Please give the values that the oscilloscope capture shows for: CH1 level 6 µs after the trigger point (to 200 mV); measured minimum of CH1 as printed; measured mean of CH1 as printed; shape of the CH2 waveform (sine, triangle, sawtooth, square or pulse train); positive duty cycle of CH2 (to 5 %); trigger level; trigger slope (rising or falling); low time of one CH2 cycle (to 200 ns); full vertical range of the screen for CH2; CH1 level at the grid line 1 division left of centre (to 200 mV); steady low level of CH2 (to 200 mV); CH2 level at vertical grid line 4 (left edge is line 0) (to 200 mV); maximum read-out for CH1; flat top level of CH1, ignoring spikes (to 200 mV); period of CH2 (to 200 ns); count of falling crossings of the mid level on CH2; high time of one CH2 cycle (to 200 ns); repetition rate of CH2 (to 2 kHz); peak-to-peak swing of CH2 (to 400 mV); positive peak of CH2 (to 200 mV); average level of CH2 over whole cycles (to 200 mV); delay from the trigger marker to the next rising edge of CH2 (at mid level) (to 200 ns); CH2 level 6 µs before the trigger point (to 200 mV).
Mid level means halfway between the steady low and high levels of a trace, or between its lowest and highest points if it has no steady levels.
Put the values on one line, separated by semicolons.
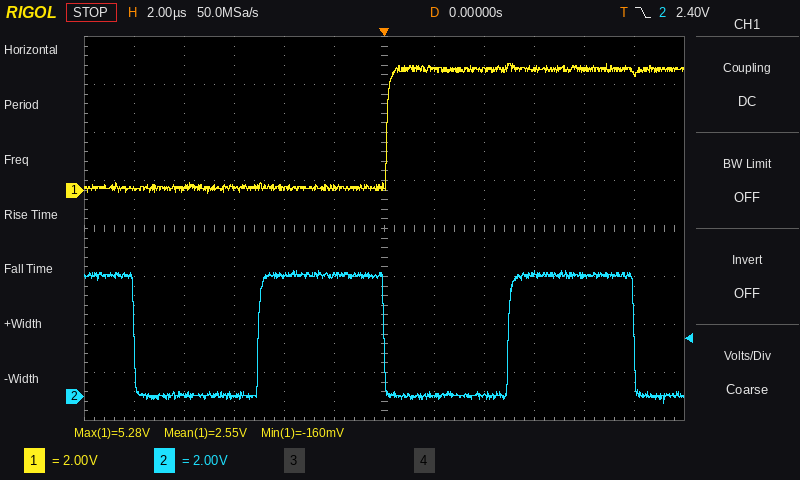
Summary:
5.0 V; -160 mV; 2.55 V; square; 50 %; 2.40 V; falling; 5.0 µs; 16 V; 200 mV; 0.0 V; 5.0 V; 5.28 V; 5.0 V; 10.0 µs; 3; 5.0 µs; 100 kHz; 5.6 V; 5.2 V; 2.6 V; 5.0 µs; 0.0 V
